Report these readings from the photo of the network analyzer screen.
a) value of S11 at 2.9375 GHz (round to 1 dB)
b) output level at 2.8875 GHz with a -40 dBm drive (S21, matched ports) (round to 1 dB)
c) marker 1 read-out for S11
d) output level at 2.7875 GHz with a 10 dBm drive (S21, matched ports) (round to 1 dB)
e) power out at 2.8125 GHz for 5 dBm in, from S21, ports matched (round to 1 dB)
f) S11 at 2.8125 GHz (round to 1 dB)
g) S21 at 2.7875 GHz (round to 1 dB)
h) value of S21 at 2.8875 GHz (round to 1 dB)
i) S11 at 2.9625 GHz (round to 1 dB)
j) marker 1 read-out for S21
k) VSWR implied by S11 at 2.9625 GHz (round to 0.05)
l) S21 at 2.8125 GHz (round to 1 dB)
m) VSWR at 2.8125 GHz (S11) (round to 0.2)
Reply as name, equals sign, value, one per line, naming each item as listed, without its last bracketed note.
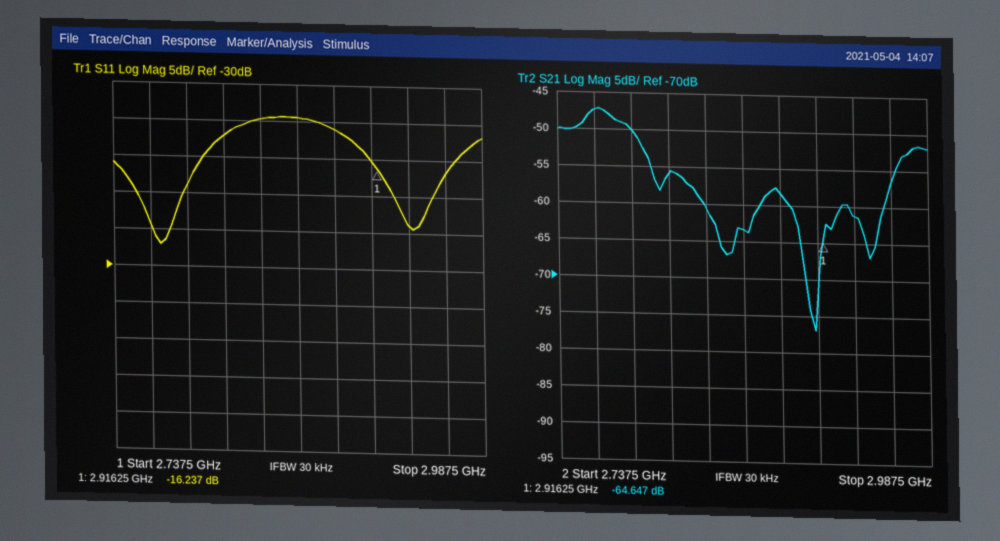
value of S11 at 2.9375 GHz = -24 dB
output level at 2.8875 GHz with a -40 dBm drive (S21, matched ports) = -98 dBm
marker 1 read-out for S11 = -16.237 dB
output level at 2.7875 GHz with a 10 dBm drive (S21, matched ports) = -40 dBm
power out at 2.8125 GHz for 5 dBm in, from S21, ports matched = -51 dBm
S11 at 2.8125 GHz = -12 dB
S21 at 2.7875 GHz = -50 dB
value of S21 at 2.8875 GHz = -58 dB
S11 at 2.9625 GHz = -17 dB
marker 1 read-out for S21 = -64.647 dB
VSWR implied by S11 at 2.9625 GHz = 1.35
S21 at 2.8125 GHz = -56 dB
VSWR at 2.8125 GHz (S11) = 1.6
